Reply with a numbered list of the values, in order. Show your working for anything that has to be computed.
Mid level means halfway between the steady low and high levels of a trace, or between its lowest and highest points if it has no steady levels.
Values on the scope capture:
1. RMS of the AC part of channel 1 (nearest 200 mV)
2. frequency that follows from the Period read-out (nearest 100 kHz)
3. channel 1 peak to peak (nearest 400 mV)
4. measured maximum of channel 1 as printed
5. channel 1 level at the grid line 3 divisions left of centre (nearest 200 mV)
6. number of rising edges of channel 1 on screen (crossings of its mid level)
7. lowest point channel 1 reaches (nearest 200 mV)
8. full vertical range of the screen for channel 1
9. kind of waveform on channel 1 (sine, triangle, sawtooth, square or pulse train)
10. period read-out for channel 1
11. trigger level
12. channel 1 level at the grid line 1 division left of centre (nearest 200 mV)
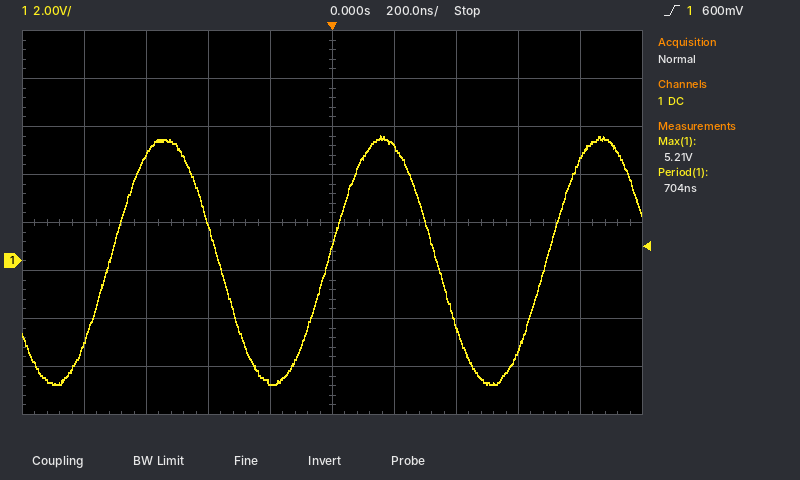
1. 10.4 V / (2√2) ≈ 3.68 V, so 3.6 V to the nearest 200 mV
2. 1 / 704 ns ≈ 1.4 MHz
3. 10.4 V
4. 5.21 V
5. 4.4 V
6. 3
7. -5.2 V
8. 16 V
9. sine
10. 704 ns
11. 600 mV
12. -5.0 V
